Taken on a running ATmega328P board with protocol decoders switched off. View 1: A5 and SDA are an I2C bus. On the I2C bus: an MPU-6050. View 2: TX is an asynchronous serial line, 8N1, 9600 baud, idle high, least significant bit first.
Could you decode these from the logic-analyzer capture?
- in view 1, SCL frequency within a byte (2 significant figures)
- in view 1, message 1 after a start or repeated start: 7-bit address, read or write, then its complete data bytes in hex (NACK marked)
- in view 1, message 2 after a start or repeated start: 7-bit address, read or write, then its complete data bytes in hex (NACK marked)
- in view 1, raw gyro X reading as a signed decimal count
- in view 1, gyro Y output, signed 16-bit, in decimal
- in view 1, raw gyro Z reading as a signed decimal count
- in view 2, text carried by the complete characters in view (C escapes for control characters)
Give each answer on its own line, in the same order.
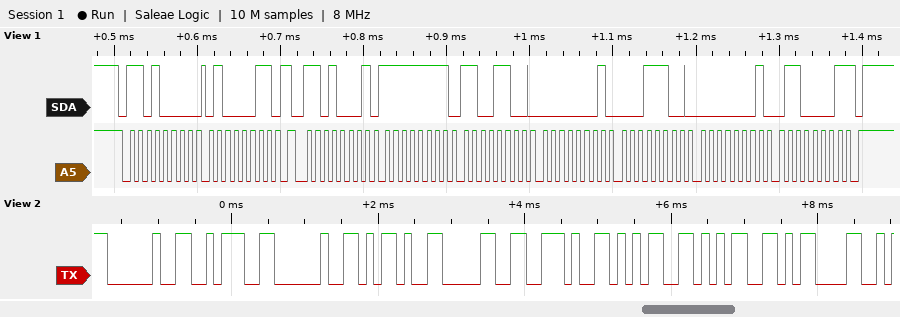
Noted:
100 kHz
0x68 write: 43
0x68 read: FF CC 01 1C 01 61 NACK
-52
284
353
" : -0.55\r"
